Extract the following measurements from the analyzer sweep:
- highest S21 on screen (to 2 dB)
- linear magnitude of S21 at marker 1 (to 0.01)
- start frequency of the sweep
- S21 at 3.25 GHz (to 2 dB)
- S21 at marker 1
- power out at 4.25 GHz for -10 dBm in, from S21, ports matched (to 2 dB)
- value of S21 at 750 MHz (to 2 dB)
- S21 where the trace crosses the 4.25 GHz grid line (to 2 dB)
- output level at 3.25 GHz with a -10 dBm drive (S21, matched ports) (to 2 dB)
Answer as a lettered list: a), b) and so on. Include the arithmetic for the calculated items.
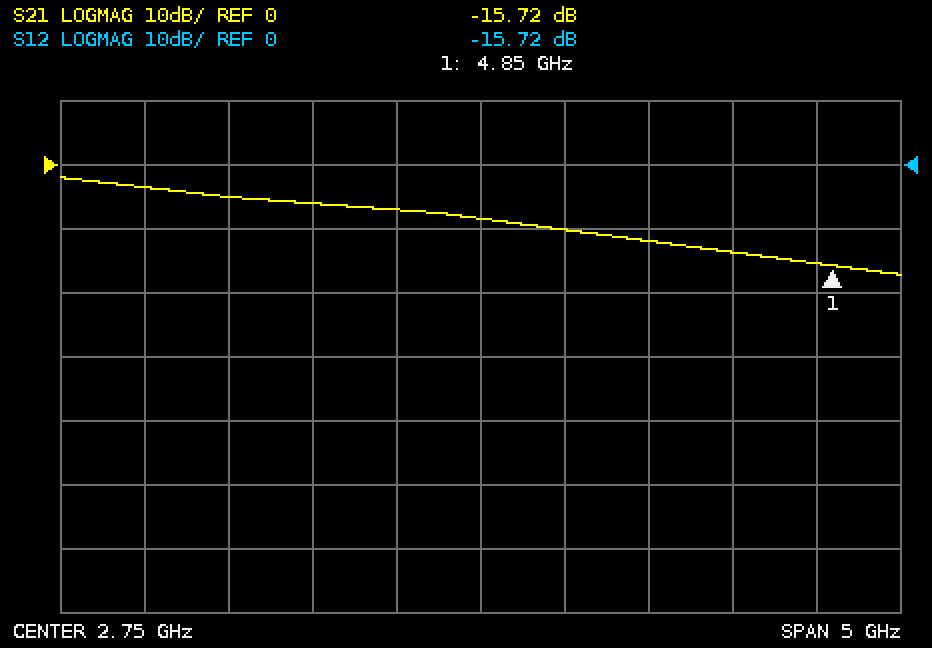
a) -2 dB
b) 10^(-15.72/20) ≈ 0.16
c) 250 MHz
d) -10 dB
e) -15.72 dB
f) -10 dBm + (-14 dB) = -24 dBm
g) -4 dB
h) -14 dB
i) -10 dBm + (-10 dB) = -20 dBm
